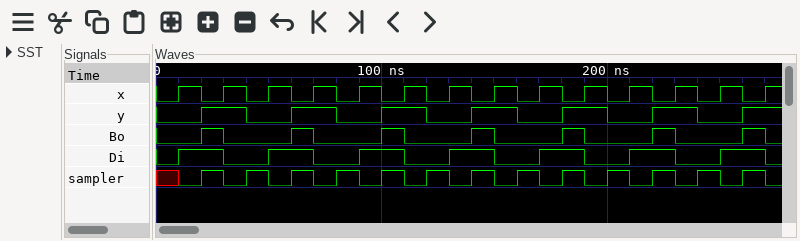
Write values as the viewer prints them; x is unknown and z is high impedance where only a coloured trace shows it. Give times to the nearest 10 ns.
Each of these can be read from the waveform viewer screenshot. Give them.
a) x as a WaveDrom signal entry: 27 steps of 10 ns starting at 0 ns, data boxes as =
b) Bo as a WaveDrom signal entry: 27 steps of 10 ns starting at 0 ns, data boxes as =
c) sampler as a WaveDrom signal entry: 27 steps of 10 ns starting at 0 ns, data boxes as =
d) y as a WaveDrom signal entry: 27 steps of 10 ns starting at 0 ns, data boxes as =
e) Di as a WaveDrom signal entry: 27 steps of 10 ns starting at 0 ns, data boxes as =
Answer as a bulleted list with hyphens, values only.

- {name: 'x', wave: '010101010101010101010101010'}
- {name: 'Bo', wave: '0.10..10..10..10..10..10..1'}
- {name: 'sampler', wave: 'x01010101010101010101010101'}
- {name: 'y', wave: '0.1.0.1.0.1.0.1.0.1.0.1.0.1'}
- {name: 'Di', wave: '01.0.1.0.1.0.1.0.1.0.1.0.1.'}
